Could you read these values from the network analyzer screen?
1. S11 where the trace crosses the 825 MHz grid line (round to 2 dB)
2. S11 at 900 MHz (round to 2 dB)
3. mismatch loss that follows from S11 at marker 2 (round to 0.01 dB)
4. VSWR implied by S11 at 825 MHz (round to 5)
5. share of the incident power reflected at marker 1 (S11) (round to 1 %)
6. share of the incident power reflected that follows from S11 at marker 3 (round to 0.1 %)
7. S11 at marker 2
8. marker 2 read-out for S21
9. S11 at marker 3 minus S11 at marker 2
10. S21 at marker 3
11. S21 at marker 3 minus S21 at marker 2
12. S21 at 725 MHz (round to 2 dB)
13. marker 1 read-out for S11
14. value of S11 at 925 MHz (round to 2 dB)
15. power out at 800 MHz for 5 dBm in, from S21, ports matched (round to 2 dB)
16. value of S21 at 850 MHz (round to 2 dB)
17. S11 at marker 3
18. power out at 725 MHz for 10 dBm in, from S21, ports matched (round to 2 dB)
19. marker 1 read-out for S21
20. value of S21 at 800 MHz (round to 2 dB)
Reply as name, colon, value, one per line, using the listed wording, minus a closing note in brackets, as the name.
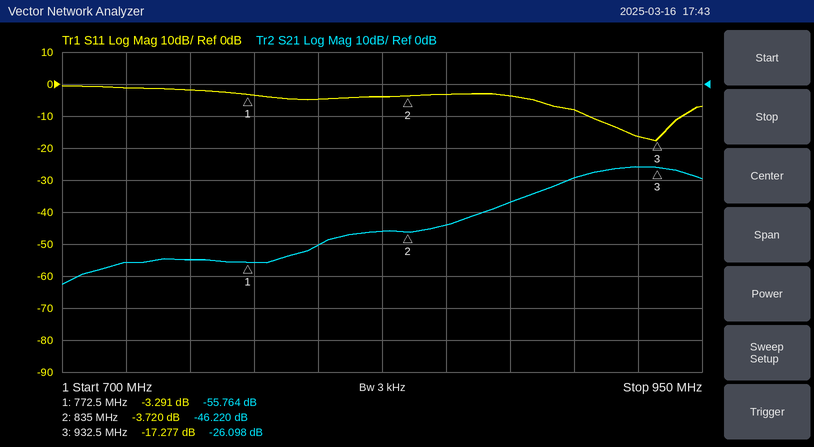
S11 where the trace crosses the 825 MHz grid line: -4 dB
S11 at 900 MHz: -8 dB
mismatch loss that follows from S11 at marker 2: 2.40 dB
VSWR implied by S11 at 825 MHz: 5
share of the incident power reflected at marker 1 (S11): 47 %
share of the incident power reflected that follows from S11 at marker 3: 1.9 %
S11 at marker 2: -3.720 dB
marker 2 read-out for S21: -46.220 dB
S11 at marker 3 minus S11 at marker 2: -13.557 dB
S21 at marker 3: -26.098 dB
S21 at marker 3 minus S21 at marker 2: 20.122 dB
S21 at 725 MHz: -56 dB
marker 1 read-out for S11: -3.291 dB
value of S11 at 925 MHz: -16 dB
power out at 800 MHz for 5 dBm in, from S21, ports matched: -46 dBm
value of S21 at 850 MHz: -44 dB
S11 at marker 3: -17.277 dB
power out at 725 MHz for 10 dBm in, from S21, ports matched: -46 dBm
marker 1 read-out for S21: -55.764 dB
value of S21 at 800 MHz: -50 dB
